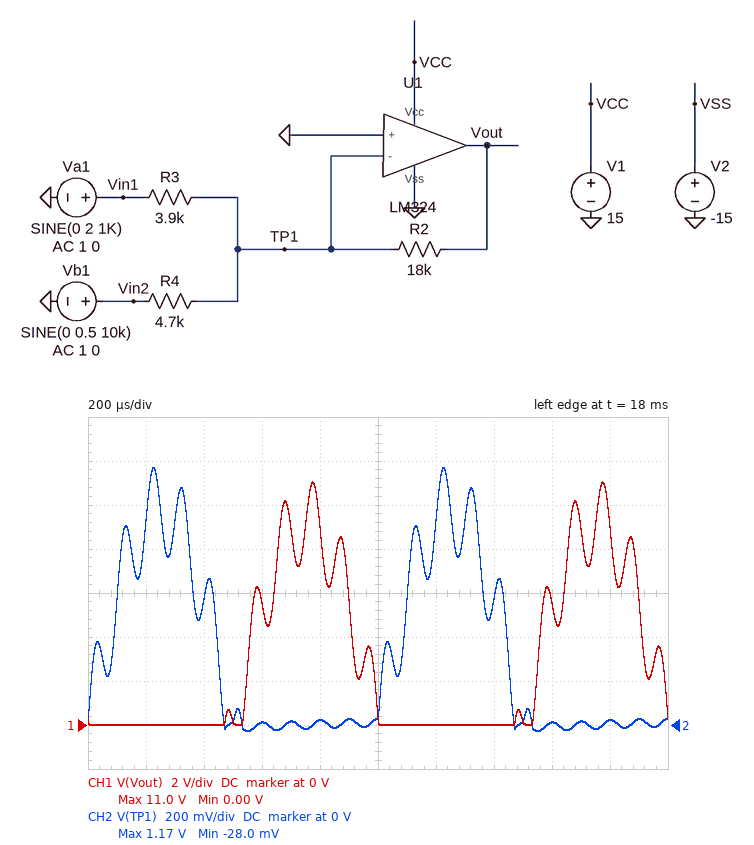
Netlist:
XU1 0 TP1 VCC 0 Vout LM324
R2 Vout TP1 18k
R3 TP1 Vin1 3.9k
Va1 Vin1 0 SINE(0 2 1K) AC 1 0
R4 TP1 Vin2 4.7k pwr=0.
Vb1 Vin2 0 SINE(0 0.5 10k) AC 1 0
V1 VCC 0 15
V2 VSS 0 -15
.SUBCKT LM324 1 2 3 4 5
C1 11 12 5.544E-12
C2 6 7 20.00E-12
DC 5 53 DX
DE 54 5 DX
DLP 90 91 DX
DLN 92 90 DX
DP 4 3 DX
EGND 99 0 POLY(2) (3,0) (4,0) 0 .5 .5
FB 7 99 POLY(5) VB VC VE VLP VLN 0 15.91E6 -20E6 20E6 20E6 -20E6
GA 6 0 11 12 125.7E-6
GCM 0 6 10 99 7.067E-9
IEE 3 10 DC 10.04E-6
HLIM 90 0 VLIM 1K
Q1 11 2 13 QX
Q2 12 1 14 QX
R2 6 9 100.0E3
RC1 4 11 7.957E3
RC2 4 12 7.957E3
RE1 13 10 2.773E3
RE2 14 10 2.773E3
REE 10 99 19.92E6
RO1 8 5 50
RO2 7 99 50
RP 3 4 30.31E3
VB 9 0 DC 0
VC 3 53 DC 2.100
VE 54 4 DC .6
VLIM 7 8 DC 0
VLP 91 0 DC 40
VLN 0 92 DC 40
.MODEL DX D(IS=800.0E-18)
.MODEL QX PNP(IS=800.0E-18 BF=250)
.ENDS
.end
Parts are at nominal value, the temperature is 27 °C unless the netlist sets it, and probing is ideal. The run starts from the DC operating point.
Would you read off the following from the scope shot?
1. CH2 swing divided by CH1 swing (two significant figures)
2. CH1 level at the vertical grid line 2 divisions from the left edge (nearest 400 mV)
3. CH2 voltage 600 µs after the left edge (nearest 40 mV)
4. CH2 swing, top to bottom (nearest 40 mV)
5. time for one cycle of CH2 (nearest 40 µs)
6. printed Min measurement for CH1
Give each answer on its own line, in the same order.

0.11
0 V
0 V
1.20 V
1.00 ms
0.00 V
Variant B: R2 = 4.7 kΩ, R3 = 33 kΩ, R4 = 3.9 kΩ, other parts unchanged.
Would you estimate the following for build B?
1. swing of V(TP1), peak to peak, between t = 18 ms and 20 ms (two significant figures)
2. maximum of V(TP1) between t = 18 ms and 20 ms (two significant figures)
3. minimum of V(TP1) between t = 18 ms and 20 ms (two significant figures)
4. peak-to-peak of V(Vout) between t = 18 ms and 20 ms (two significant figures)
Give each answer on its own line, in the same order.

390 mV
380 mV
-16 mV
880 mV
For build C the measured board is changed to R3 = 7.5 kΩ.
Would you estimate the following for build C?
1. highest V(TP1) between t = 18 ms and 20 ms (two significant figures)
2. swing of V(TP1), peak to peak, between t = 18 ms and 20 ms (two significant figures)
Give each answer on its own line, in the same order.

920 mV
950 mV
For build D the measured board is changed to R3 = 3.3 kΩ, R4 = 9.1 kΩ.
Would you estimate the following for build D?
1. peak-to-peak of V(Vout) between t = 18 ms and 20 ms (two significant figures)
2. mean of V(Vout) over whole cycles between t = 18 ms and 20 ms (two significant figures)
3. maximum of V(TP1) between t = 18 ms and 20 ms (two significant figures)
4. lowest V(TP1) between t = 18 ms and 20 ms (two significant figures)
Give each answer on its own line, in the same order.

12 V
3.5 V
1.4 V
-20 mV
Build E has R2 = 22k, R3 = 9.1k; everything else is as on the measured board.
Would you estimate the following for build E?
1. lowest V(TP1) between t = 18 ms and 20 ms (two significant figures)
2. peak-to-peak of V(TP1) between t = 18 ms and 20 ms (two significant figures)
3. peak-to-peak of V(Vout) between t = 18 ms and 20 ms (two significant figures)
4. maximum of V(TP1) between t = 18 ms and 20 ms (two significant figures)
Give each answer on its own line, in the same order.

-34 mV
910 mV
7.1 V
880 mV
